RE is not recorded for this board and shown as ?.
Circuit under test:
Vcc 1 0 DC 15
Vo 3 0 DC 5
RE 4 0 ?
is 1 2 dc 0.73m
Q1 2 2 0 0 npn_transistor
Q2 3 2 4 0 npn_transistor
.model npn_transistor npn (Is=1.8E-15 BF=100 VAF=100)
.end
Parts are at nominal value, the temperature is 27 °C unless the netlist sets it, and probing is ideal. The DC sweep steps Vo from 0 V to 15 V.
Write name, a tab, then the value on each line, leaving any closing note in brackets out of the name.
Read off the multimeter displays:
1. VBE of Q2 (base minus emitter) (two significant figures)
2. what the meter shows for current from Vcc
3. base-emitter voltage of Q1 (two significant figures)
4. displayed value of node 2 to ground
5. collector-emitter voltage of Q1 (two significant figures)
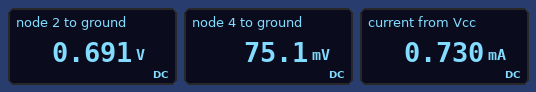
VBE of Q2 (base minus emitter)	620 mV
what the meter shows for current from Vcc	0.730 mA
base-emitter voltage of Q1	690 mV
displayed value of node 2 to ground	0.691 V
collector-emitter voltage of Q1	690 mV
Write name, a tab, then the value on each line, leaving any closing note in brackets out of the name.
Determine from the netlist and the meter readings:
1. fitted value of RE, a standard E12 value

fitted value of RE, a standard E12 value	1.8 kΩ
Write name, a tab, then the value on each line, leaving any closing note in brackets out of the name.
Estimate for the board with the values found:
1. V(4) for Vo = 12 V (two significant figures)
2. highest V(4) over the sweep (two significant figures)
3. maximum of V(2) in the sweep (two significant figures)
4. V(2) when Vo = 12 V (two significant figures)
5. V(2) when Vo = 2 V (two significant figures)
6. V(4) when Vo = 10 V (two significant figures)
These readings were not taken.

V(4) for Vo = 12 V	76 mV
highest V(4) over the sweep	77 mV
maximum of V(2) in the sweep	690 mV
V(2) when Vo = 12 V	690 mV
V(2) when Vo = 2 V	690 mV
V(4) when Vo = 10 V	76 mV
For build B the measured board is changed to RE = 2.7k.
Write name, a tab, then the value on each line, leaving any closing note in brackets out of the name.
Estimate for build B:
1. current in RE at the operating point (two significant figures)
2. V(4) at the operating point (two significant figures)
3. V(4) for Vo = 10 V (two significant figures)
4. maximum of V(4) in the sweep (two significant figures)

current in RE at the operating point	31 µA
V(4) at the operating point	83 mV
V(4) for Vo = 10 V	84 mV
maximum of V(4) in the sweep	85 mV
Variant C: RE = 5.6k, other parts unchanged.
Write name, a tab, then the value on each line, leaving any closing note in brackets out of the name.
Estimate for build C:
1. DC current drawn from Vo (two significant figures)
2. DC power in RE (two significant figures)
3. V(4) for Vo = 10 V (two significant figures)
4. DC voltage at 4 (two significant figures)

DC current drawn from Vo	17 µA
DC power in RE	1.7 µW
V(4) for Vo = 10 V	99 mV
DC voltage at 4	98 mV
